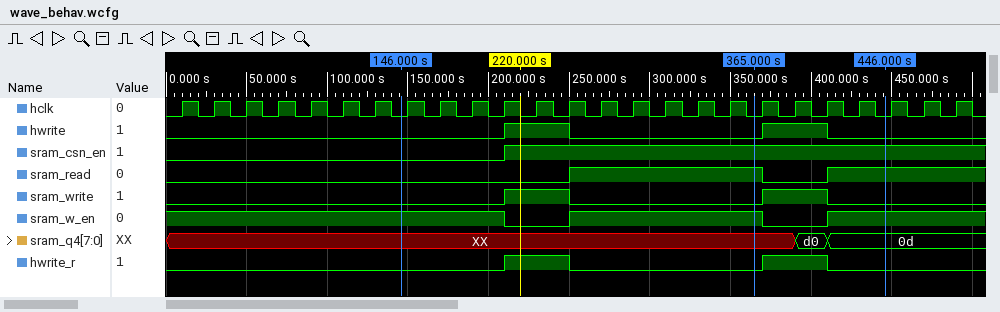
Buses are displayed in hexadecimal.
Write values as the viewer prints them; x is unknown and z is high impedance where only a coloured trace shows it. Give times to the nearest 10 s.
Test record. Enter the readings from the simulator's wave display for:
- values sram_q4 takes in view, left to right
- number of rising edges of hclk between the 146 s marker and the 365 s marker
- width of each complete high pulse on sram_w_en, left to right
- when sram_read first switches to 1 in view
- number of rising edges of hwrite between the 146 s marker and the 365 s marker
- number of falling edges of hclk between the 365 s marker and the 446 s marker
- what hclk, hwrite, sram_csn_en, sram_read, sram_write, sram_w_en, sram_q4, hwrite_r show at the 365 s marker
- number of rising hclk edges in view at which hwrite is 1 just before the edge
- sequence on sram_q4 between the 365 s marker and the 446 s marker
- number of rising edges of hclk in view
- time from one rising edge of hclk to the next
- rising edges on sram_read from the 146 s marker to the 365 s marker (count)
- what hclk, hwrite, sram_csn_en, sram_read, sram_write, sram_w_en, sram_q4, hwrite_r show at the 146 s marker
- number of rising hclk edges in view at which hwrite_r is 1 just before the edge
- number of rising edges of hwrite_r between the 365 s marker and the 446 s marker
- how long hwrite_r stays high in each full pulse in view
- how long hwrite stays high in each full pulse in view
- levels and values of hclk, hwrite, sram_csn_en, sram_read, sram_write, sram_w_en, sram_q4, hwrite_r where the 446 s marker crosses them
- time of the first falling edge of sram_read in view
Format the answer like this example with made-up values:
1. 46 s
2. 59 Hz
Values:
1. XX, d0, 0d
2. 11
3. 120 s
4. 250 s
5. 1
6. 4
7. hclk=0, hwrite=0, sram_csn_en=1, sram_read=1, sram_write=0, sram_w_en=1, sram_q4=XX, hwrite_r=0
8. 4
9. XX, d0, 0d
10. 25
11. 20 s
12. 1
13. hclk=0, hwrite=0, sram_csn_en=0, sram_read=0, sram_write=0, sram_w_en=1, sram_q4=XX, hwrite_r=0
14. 4
15. 1
16. 40 s, 40 s
17. 40 s, 40 s
18. hclk=0, hwrite=0, sram_csn_en=1, sram_read=1, sram_write=0, sram_w_en=1, sram_q4=0d, hwrite_r=0
19. 370 s
